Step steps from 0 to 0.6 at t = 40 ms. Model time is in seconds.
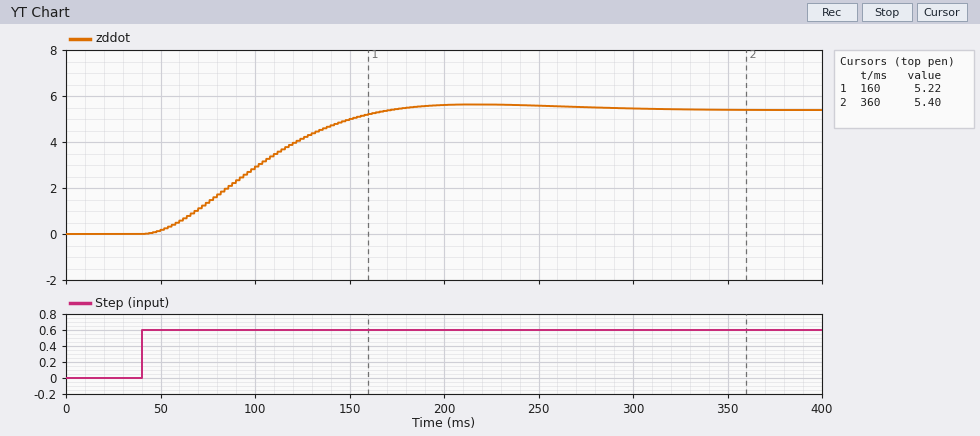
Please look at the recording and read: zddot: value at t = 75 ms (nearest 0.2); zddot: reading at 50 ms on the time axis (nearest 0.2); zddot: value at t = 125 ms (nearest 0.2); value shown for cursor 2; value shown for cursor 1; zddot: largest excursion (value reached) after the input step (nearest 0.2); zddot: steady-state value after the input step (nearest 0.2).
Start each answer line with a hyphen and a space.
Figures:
- 1.4
- 0.2
- 4.2
- 5.40
- 5.22
- 5.6
- 5.4
